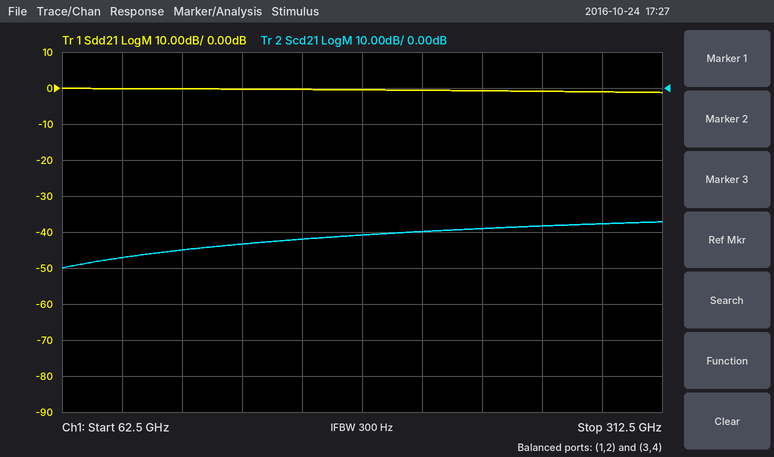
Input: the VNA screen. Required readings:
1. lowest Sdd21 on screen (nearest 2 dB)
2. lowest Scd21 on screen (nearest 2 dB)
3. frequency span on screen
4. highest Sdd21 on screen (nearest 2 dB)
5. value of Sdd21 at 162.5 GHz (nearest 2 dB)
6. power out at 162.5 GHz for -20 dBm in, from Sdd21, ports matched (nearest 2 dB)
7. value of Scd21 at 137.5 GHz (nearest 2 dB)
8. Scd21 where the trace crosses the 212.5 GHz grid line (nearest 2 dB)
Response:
-2 dB
-50 dB
250 GHz
0 dB
0 dB
-20 dBm
-44 dB
-40 dB
